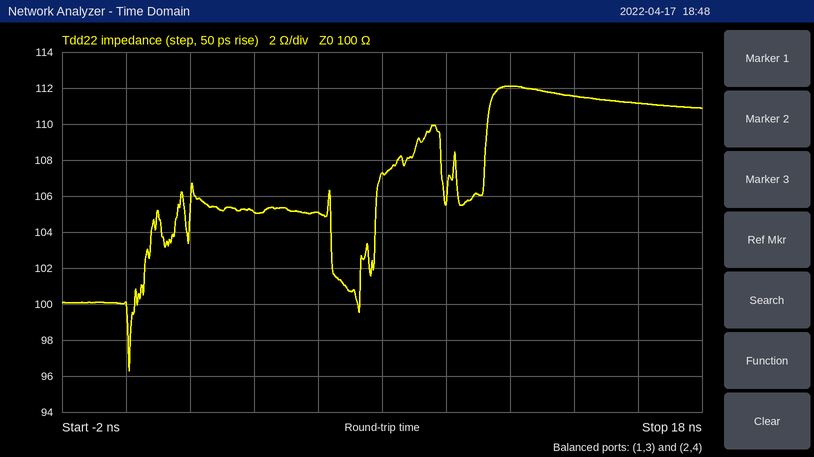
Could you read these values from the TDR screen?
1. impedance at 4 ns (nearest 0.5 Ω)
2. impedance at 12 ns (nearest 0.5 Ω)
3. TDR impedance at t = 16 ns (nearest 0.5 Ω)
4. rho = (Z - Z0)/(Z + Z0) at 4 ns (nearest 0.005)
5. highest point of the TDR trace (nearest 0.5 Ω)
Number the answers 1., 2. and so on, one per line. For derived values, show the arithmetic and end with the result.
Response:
1. 105.0 Ω
2. 112.0 Ω
3. 111.0 Ω
4. (105 − 100)/(105 + 100) ≈ +0.0244, so +0.025 to the nearest 0.005
5. 112.0 Ω
